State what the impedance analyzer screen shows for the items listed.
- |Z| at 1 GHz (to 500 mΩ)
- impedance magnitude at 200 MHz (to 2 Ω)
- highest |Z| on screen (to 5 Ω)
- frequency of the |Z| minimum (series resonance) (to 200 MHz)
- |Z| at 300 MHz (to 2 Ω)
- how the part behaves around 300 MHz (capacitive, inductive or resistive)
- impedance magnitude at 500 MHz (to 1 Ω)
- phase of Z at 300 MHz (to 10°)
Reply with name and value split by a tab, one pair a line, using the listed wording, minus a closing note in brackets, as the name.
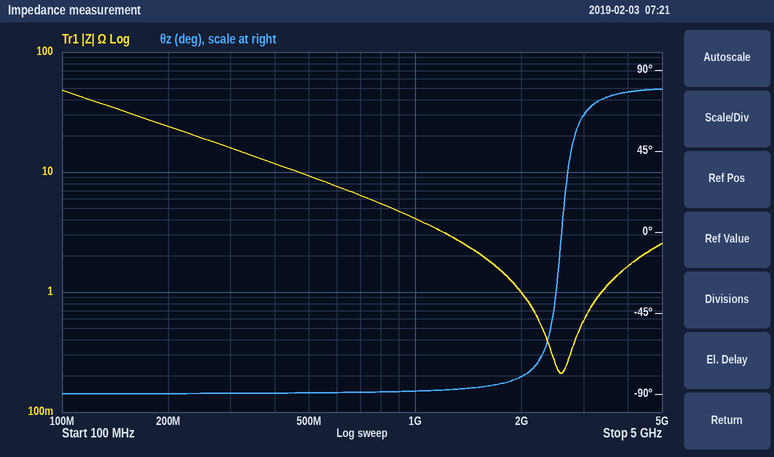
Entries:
|Z| at 1 GHz	4.0 Ω
impedance magnitude at 200 MHz	24 Ω
highest |Z| on screen	50 Ω
frequency of the |Z| minimum (series resonance)	2.6 GHz
|Z| at 300 MHz	16 Ω
how the part behaves around 300 MHz	capacitive
impedance magnitude at 500 MHz	9 Ω
phase of Z at 300 MHz	-90°
